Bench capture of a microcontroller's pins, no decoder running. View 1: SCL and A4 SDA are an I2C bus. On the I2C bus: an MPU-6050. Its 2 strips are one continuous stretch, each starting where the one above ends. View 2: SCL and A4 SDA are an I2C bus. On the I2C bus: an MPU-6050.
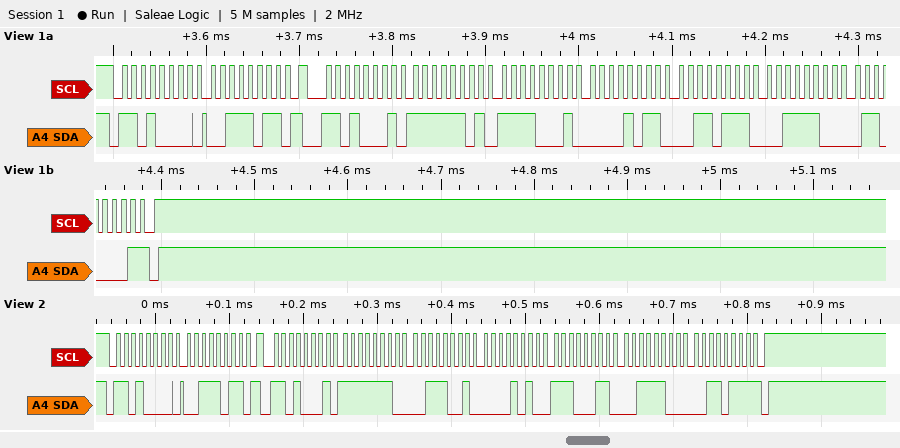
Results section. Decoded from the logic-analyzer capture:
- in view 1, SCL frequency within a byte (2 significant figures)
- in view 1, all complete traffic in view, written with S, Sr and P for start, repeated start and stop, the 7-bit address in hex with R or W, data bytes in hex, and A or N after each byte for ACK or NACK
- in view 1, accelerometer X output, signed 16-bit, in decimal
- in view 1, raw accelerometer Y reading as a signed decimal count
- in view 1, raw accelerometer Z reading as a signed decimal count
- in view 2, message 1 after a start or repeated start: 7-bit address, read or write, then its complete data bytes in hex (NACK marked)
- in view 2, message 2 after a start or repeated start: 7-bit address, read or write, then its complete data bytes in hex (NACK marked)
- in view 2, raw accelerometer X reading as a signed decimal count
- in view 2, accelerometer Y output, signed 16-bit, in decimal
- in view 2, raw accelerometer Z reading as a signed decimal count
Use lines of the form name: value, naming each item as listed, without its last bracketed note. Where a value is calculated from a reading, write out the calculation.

in view 1, SCL frequency within a byte: 100 kHz
in view 1, all complete traffic in view, written with S, Sr and P for start, repeated start and stop, the 7-bit address in hex with R or W, data bytes in hex, and A or N after each byte for ACK or NACK: S 68W A 3B A Sr 68R A FD A F1 A 0B A 37 A 3C A 61 N P
in view 1, accelerometer X output, signed 16-bit, in decimal: 0xFDF1 = -527
in view 1, raw accelerometer Y reading as a signed decimal count: 0x0B37 = 2871
in view 1, raw accelerometer Z reading as a signed decimal count: 0x3C61 = 15457
in view 2, message 1 after a start or repeated start: 7-bit address, read or write, then its complete data bytes in hex: 0x68 write: 3B
in view 2, message 2 after a start or repeated start: 7-bit address, read or write, then its complete data bytes in hex: 0x68 read: FE 39 0A E3 3C 37 NACK
in view 2, raw accelerometer X reading as a signed decimal count: 0xFE39 = -455
in view 2, accelerometer Y output, signed 16-bit, in decimal: 0x0AE3 = 2787
in view 2, raw accelerometer Z reading as a signed decimal count: 0x3C37 = 15415
